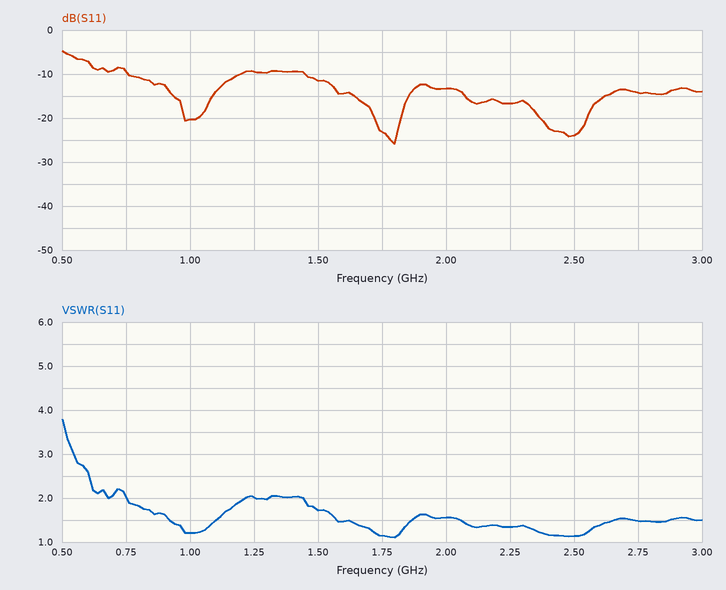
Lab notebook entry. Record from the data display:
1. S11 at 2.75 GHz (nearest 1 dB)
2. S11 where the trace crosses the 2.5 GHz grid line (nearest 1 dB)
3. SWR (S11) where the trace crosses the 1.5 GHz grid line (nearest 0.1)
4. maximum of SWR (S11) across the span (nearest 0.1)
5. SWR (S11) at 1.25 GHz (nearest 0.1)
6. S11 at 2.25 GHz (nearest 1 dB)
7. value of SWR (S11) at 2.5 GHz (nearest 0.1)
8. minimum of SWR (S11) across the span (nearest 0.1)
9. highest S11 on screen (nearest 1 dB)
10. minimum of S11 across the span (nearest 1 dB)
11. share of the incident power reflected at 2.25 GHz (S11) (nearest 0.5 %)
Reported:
-14 dB
-24 dB
1.7
3.8
2.0
-17 dB
1.1
1.1
-5 dB
-26 dB
2.0 %
